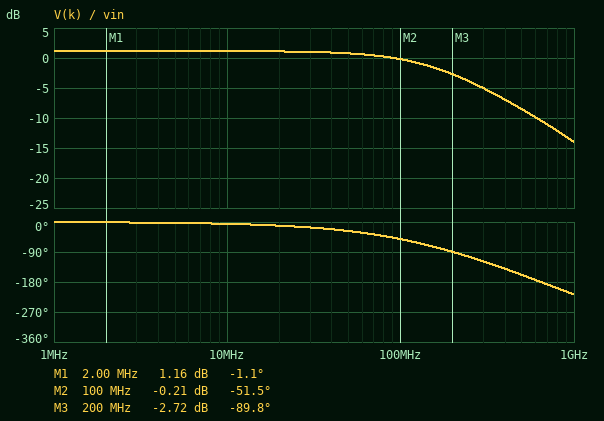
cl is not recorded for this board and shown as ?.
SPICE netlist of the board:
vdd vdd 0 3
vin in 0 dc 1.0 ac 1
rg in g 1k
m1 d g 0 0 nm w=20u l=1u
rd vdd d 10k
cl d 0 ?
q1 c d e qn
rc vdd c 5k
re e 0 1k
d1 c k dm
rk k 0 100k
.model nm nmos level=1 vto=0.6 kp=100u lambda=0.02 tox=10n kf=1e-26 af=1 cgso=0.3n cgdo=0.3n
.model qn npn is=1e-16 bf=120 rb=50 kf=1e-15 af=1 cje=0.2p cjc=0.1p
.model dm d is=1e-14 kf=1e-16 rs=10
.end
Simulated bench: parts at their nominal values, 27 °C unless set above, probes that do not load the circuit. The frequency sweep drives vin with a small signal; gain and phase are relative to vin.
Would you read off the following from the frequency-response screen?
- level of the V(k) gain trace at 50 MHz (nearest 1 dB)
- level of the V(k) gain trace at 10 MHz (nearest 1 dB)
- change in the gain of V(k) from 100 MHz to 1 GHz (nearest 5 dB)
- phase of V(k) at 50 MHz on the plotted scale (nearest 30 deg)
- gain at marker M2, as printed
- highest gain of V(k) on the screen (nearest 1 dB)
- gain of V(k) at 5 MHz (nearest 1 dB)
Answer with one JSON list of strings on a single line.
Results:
["1 dB", "1 dB", "-15 dB", "-30 deg", "-0.21 dB", "1 dB", "1 dB"]
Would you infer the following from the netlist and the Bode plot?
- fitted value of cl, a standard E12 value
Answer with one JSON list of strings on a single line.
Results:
["470 fF"]
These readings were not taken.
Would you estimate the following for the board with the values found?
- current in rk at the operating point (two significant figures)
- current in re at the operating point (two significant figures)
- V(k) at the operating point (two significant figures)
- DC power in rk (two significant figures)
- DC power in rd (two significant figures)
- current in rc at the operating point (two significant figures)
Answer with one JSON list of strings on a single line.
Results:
["1.2 µA", "490 µA", "120 mV", "140 nW", "310 µW", "480 µA"]
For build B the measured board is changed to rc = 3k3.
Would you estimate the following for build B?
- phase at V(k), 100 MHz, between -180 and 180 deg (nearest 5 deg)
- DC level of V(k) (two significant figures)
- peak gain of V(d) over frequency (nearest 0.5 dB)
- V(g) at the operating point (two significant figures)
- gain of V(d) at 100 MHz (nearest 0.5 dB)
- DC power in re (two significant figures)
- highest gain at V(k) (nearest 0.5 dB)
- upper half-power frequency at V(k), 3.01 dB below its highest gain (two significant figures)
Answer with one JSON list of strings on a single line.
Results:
["-95 deg", "640 mV", "17.5 dB", "1.0 V", "3.0 dB", "310 µW", "26.5 dB", "19 MHz"]
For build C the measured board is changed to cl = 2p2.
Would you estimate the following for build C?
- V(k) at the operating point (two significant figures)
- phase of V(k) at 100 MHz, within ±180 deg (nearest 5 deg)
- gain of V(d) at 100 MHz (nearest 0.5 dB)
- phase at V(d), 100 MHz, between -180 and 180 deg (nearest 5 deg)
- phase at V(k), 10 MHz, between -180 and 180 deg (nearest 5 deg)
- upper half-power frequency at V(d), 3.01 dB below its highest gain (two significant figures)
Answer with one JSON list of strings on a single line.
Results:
["120 mV", "-85 deg", "-6.0 dB", "115 deg", "-15 deg", "49 MHz"]
